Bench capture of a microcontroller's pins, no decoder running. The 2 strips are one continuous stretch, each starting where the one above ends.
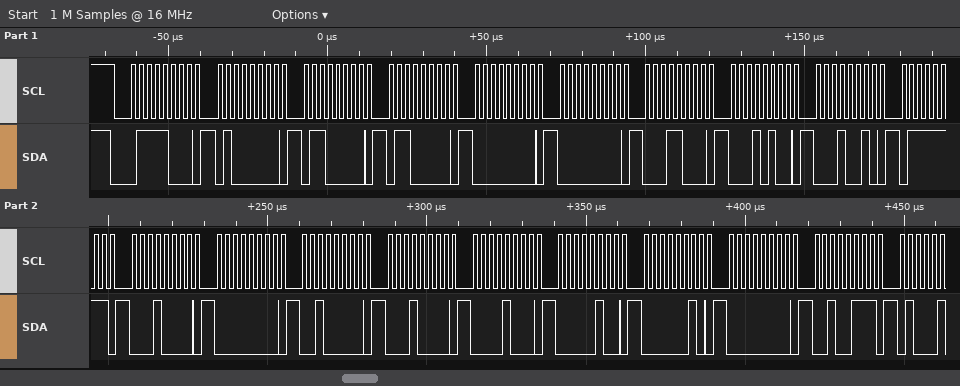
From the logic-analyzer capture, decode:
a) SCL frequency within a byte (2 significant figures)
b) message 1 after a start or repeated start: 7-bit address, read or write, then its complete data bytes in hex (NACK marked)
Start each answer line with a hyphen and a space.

- 400 kHz
- 0x3C write: 40 60 60 00 00 18 14 12 7F 10 00 20 10 08 04 02 00 27
